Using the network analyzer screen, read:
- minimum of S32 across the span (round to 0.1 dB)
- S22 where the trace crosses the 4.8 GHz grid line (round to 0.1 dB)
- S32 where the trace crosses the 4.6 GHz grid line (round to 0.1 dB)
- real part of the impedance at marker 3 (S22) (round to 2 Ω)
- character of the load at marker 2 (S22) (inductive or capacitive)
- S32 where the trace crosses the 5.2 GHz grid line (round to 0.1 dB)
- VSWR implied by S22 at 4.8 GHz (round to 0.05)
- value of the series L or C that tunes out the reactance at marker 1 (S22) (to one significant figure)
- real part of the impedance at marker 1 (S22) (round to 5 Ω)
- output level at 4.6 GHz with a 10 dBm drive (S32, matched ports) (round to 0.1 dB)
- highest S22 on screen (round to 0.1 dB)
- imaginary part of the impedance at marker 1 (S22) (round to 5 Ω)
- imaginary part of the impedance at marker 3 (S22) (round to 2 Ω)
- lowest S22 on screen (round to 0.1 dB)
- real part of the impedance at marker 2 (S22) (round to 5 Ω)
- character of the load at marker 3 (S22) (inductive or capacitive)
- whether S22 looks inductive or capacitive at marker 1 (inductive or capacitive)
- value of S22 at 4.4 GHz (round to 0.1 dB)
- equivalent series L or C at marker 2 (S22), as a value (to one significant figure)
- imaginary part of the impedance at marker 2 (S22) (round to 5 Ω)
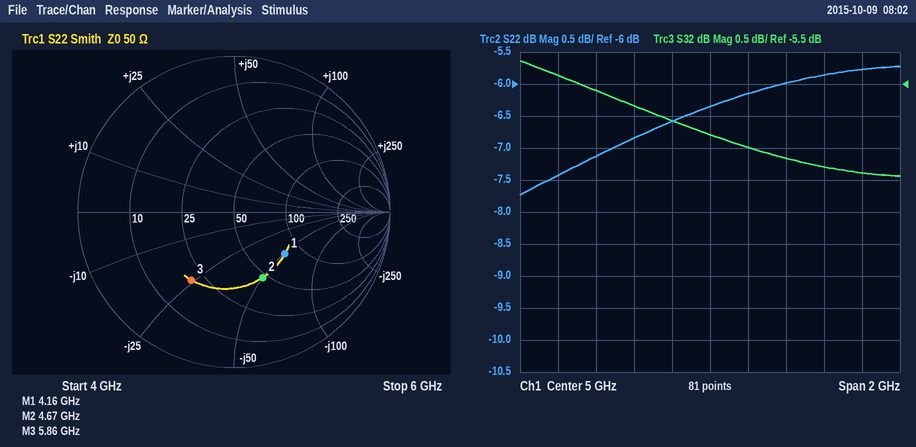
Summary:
-6.9 dB
-6.6 dB
-5.8 dB
20 Ω
capacitive
-6.5 dB
2.75
2 nH
80 Ω
4.2 dBm
-5.7 dB
-50 Ω
-24 Ω
-7.7 dB
45 Ω
capacitive
capacitive
-7.1 dB
700 fF
-50 Ω
